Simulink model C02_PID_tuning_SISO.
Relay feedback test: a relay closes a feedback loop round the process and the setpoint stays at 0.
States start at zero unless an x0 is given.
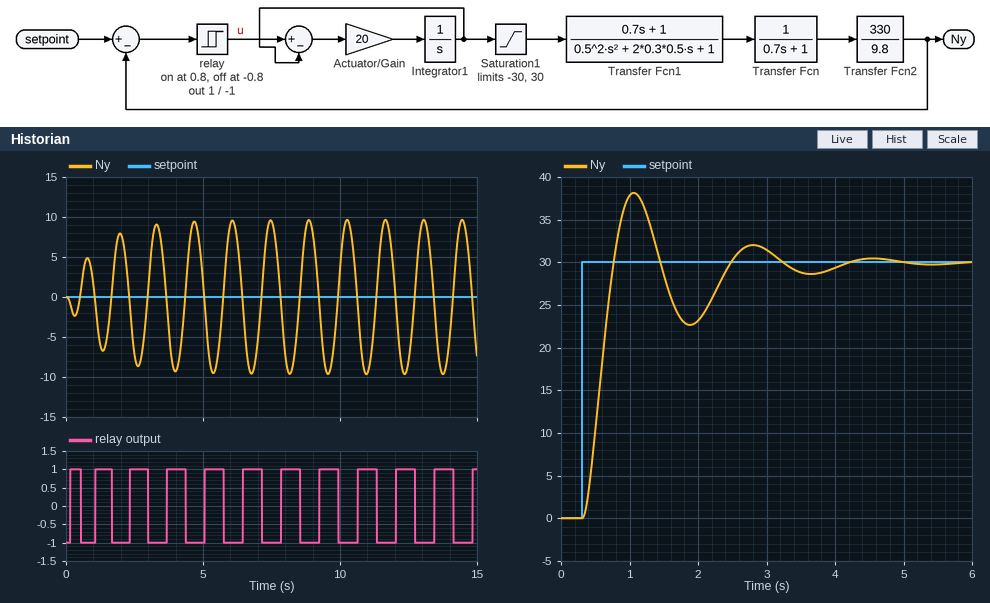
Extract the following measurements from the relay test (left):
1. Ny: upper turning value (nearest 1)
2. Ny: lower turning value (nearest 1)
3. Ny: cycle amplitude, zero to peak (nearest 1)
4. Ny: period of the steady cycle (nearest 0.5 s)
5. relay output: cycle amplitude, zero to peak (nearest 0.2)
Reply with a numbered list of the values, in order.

1. 10
2. -10
3. 10
4. 1.5 s
5. 1.0
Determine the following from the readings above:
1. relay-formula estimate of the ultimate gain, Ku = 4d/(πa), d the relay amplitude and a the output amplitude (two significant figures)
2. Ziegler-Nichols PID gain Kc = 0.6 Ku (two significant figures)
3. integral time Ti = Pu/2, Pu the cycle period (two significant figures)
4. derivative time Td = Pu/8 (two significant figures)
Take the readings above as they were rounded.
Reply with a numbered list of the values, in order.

1. 0.13
2. 0.078
3. 0.75 s
4. 0.19 s
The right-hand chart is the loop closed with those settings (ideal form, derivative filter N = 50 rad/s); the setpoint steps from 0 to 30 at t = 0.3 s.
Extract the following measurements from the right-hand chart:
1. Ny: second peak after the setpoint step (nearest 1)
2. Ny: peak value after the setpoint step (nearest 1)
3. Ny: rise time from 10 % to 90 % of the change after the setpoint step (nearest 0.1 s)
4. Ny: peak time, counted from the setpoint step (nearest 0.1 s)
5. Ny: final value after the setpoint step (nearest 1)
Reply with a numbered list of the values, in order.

1. 32
2. 38
3. 0.3 s
4. 0.8 s
5. 30
